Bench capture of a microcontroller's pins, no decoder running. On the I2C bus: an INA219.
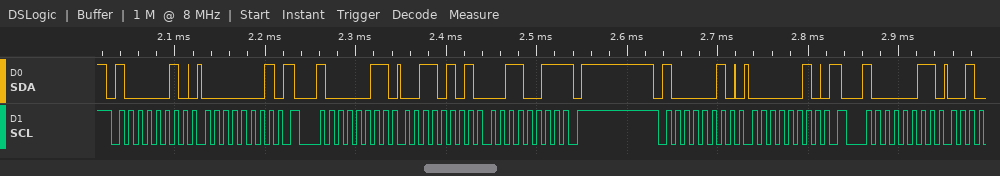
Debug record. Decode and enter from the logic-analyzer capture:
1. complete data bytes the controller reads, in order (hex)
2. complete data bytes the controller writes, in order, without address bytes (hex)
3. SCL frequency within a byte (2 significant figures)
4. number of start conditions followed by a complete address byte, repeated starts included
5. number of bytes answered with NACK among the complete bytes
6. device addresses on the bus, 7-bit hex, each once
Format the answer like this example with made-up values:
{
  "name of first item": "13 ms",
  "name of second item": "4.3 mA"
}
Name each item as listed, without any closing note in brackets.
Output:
{
  "complete data bytes the controller reads, in order": "35 33",
  "complete data bytes the controller writes, in order, without address bytes": "01 02",
  "SCL frequency within a byte": "100 kHz",
  "number of start conditions followed by a complete address byte, repeated starts included": "4",
  "number of bytes answered with NACK among the complete bytes": "1",
  "device addresses on the bus, 7-bit hex, each once": "0x41"
}
